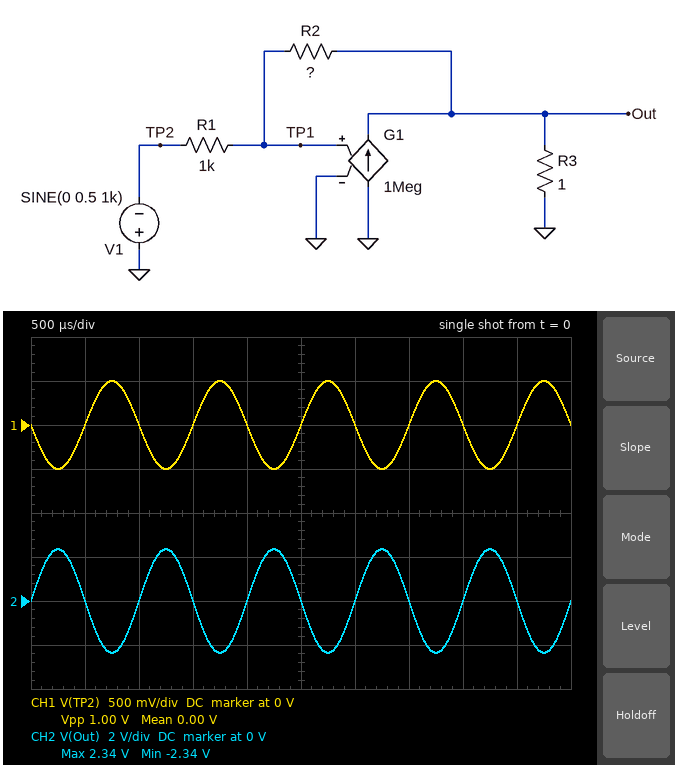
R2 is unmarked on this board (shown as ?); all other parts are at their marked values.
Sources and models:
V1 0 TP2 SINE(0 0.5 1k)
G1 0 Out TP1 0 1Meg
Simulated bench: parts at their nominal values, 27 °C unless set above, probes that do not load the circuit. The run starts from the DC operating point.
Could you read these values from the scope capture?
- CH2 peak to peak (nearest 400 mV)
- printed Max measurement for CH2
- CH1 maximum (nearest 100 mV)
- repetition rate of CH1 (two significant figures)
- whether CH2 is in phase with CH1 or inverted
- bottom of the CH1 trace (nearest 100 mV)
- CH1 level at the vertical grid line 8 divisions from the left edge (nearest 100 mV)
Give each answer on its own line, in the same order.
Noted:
4.8 V
2.34 V
500 mV
1.0 kHz
inverted
-500 mV
0 V
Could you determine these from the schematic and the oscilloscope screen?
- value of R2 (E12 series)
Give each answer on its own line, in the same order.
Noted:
4.7 kΩ
